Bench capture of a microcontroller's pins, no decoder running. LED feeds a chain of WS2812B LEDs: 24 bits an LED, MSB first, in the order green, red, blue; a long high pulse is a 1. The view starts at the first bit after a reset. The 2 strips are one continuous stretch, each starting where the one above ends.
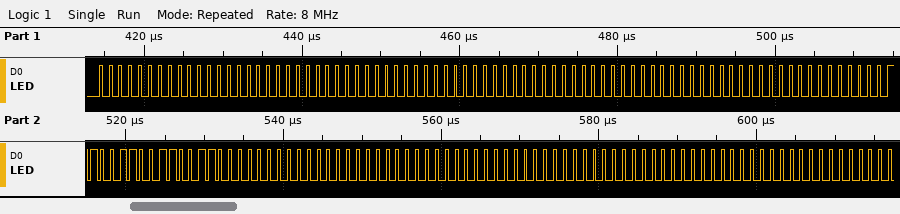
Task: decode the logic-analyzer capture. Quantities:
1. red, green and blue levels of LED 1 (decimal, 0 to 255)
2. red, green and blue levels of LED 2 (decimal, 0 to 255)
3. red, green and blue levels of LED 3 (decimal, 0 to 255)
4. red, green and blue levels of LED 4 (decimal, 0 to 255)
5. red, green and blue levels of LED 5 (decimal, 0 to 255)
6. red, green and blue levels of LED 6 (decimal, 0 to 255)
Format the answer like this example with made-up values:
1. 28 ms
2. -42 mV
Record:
1. 0, 0, 0
2. 0, 0, 0
3. 0, 0, 0
4. 204, 0, 204
5. 0, 0, 0
6. 0, 0, 0
